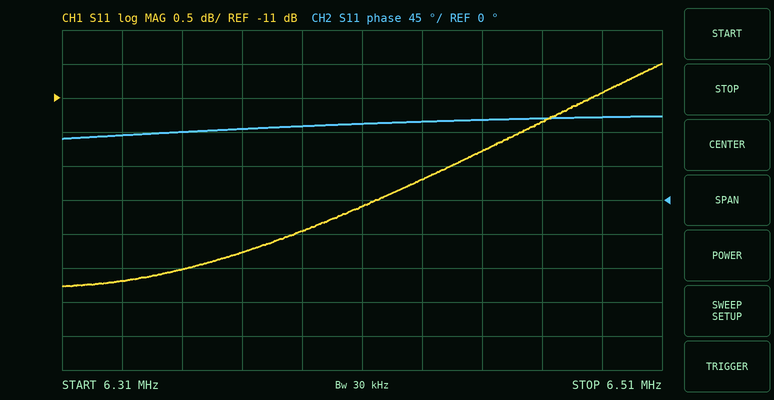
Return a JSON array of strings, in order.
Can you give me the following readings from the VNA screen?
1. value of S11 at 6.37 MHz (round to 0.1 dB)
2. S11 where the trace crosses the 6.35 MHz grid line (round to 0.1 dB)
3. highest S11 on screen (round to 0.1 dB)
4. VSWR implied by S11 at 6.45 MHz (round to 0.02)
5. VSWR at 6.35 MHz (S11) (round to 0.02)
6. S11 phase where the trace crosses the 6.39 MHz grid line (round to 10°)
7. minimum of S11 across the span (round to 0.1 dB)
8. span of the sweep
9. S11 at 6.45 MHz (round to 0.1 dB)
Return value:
["-13.3 dB", "-13.5 dB", "-10.5 dB", "1.70", "1.54", "100°", "-13.8 dB", "200 kHz", "-11.8 dB"]
